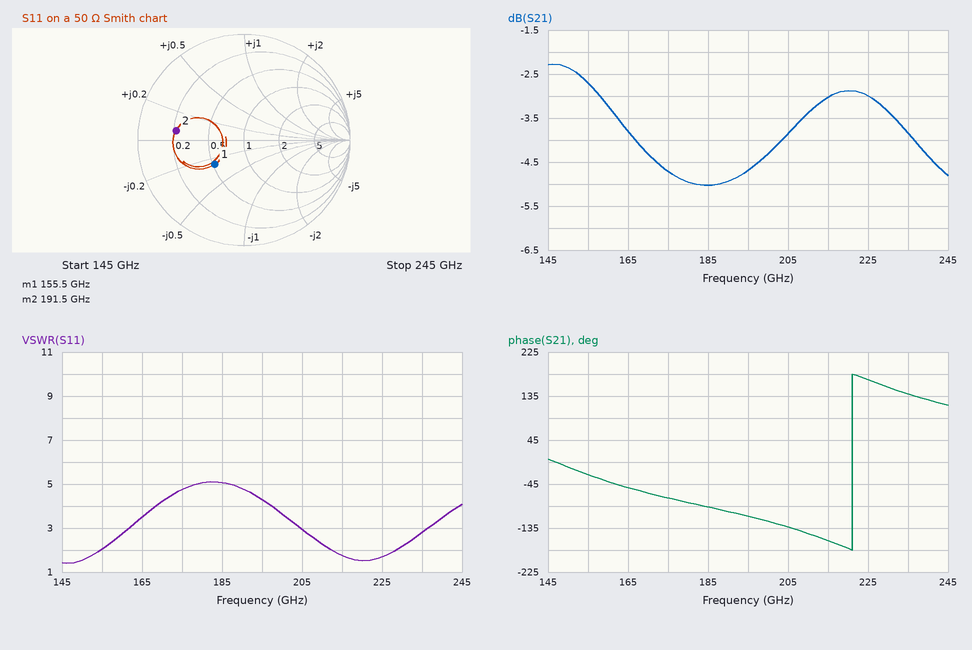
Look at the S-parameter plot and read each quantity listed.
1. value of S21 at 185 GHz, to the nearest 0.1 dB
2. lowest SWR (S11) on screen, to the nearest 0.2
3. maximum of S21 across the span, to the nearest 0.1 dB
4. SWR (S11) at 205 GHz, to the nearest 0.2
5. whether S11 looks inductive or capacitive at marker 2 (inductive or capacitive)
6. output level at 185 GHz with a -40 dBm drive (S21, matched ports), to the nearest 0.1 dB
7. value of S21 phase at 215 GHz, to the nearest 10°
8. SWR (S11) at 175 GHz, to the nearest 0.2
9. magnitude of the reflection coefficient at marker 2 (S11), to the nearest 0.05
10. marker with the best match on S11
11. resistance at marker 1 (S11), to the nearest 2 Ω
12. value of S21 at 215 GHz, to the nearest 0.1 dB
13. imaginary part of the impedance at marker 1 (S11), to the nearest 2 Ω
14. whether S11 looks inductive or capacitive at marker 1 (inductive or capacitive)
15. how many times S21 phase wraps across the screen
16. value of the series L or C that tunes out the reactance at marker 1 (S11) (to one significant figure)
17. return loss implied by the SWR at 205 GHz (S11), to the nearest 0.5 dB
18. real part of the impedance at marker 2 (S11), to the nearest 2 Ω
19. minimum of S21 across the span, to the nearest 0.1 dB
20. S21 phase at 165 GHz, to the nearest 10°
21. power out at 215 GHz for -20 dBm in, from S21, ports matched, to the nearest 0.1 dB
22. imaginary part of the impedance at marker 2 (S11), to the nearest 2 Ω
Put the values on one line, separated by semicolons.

-5.0 dB; 1.4; -2.3 dB; 3.0; inductive; -45.0 dBm; -160°; 4.8; 0.65; marker 1; 26 Ω; -3.0 dB; -14 Ω; capacitive; 1; 10 pH; 6.0 dB; 10 Ω; -5.0 dB; -50°; -23.0 dBm; +4 Ω
